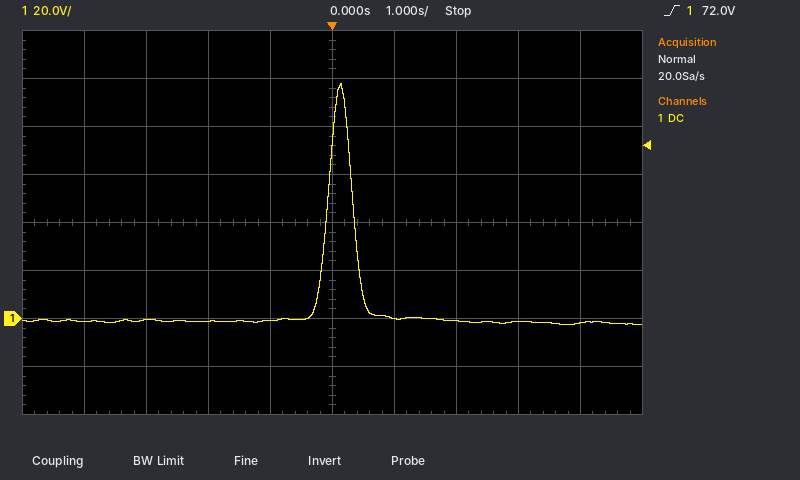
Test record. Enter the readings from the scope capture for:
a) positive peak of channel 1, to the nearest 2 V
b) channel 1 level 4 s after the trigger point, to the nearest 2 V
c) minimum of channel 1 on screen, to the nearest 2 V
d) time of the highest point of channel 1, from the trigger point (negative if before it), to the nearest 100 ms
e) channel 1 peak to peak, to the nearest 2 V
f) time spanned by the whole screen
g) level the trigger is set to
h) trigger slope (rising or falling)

98 V
-2 V
-2 V
+100 ms
100 V
10 s
72.0 V
rising
